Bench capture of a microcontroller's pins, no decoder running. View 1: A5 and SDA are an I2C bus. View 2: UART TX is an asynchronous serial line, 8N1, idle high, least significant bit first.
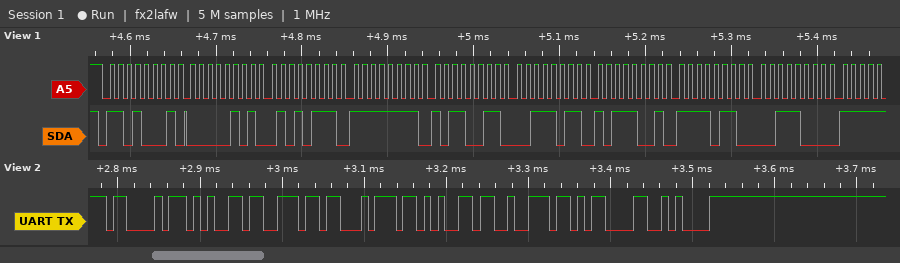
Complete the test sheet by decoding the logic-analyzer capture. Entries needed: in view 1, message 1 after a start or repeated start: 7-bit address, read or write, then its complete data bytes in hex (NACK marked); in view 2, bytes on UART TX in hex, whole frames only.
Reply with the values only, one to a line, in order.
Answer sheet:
0x68 read: 05 57 FF B3 3B B9 F6 38
43 65 6E 74 65 72 0D 0A
